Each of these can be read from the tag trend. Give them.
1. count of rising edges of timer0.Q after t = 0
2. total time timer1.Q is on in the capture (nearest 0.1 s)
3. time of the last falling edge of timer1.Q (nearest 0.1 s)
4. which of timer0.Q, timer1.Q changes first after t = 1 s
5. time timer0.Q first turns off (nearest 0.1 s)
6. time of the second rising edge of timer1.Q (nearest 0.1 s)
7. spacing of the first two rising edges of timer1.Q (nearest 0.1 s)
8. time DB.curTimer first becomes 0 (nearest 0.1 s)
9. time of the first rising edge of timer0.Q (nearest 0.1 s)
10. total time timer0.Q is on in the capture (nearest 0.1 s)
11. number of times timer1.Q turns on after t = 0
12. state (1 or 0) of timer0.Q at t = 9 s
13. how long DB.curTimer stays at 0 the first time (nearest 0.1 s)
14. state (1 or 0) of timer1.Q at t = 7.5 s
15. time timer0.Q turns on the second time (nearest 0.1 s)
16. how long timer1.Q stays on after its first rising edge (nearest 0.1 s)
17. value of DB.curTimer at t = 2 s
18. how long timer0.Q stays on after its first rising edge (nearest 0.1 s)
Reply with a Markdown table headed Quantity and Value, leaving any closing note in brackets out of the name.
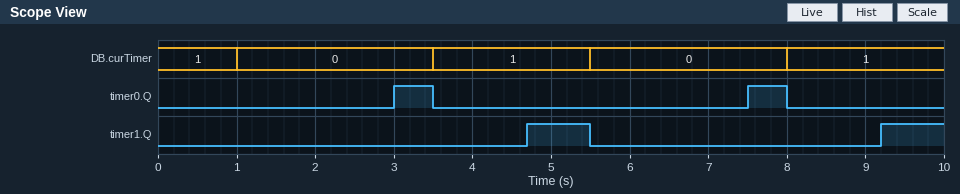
| Quantity | Value |
|---|---|
| count of rising edges of timer0.Q after t = 0 | 2 |
| total time timer1.Q is on in the capture | 1.6 s |
| time of the last falling edge of timer1.Q | 5.5 s |
| which of timer0.Q, timer1.Q changes first after t = 1 s | timer0.Q |
| time timer0.Q first turns off | 3.5 s |
| time of the second rising edge of timer1.Q | 9.2 s |
| spacing of the first two rising edges of timer1.Q | 4.5 s |
| time DB.curTimer first becomes 0 | 1.0 s |
| time of the first rising edge of timer0.Q | 3.0 s |
| total time timer0.Q is on in the capture | 1.0 s |
| number of times timer1.Q turns on after t = 0 | 2 |
| state (1 or 0) of timer0.Q at t = 9 s | 0 |
| how long DB.curTimer stays at 0 the first time | 2.5 s |
| state (1 or 0) of timer1.Q at t = 7.5 s | 0 |
| time timer0.Q turns on the second time | 7.5 s |
| how long timer1.Q stays on after its first rising edge | 0.8 s |
| value of DB.curTimer at t = 2 s | 0 |
| how long timer0.Q stays on after its first rising edge | 0.5 s |
